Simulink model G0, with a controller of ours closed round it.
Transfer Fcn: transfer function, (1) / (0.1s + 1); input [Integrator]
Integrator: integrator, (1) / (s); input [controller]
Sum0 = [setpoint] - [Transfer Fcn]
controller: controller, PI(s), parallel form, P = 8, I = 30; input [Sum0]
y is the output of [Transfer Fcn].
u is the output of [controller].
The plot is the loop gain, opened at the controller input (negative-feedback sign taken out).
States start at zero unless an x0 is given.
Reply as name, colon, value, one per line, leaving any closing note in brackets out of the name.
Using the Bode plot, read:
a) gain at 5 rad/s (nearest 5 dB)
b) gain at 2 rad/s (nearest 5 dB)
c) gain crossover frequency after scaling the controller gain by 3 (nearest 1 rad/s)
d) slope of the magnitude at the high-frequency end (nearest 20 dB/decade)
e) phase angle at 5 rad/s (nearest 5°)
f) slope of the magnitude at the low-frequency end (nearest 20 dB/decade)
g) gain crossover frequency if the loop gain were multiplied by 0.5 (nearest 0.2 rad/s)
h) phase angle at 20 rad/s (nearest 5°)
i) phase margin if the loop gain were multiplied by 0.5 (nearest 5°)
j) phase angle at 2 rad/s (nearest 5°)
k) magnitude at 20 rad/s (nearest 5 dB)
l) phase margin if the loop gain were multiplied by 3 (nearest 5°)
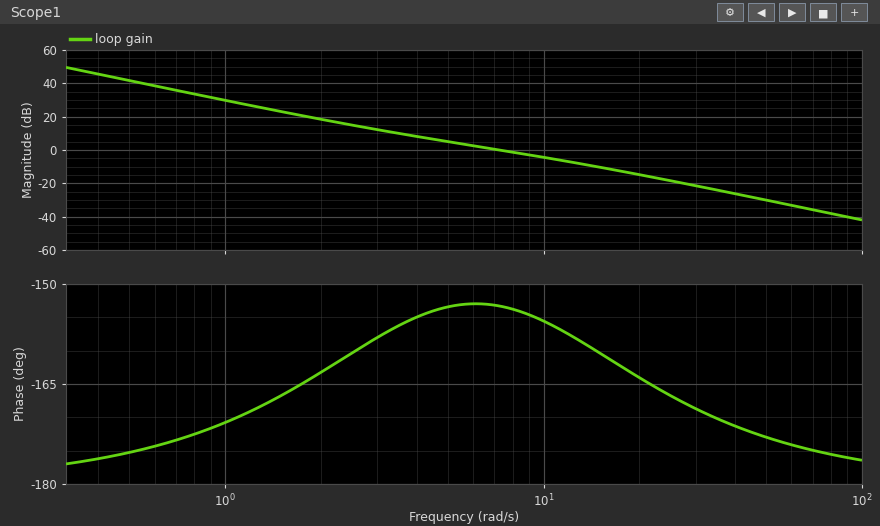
gain at 5 rad/s: 5 dB
gain at 2 rad/s: 20 dB
gain crossover frequency after scaling the controller gain by 3: 14 rad/s
slope of the magnitude at the high-frequency end: -40 dB/decade
phase angle at 5 rad/s: -155°
slope of the magnitude at the low-frequency end: -40 dB/decade
gain crossover frequency if the loop gain were multiplied by 0.5: 4.6 rad/s
phase angle at 20 rad/s: -165°
phase margin if the loop gain were multiplied by 0.5: 25°
phase angle at 2 rad/s: -165°
magnitude at 20 rad/s: -15 dB
phase margin if the loop gain were multiplied by 3: 20°
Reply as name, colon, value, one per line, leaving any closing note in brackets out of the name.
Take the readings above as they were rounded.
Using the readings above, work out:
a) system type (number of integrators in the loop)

system type: 2
